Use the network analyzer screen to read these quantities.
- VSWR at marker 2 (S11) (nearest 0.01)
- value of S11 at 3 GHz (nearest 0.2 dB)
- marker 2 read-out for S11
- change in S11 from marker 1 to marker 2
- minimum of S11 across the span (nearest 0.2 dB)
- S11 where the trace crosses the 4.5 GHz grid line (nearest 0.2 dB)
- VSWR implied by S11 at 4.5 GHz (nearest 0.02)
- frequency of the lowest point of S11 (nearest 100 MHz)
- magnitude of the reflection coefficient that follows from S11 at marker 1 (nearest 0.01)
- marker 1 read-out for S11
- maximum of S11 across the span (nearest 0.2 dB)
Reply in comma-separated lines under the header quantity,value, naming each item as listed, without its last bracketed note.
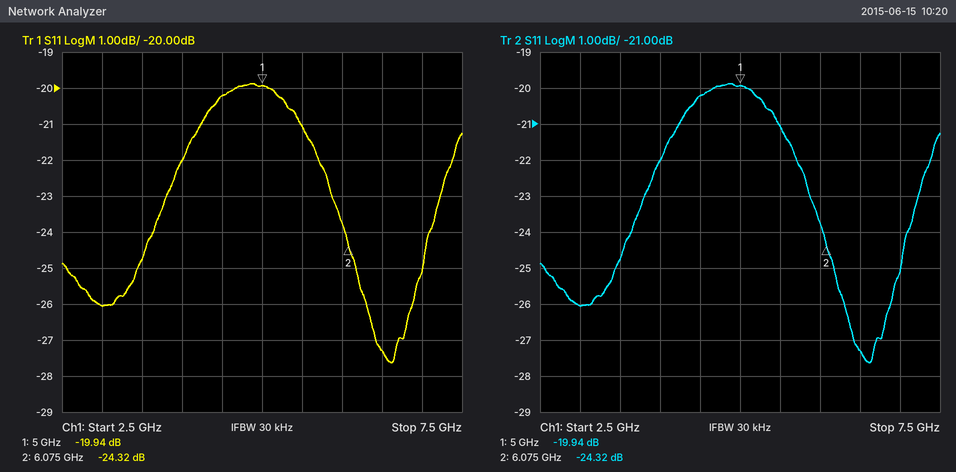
quantity,value
VSWR at marker 2 (S11),1.13
value of S11 at 3 GHz,-26.0 dB
marker 2 read-out for S11,-24.32 dB
change in S11 from marker 1 to marker 2,-4.38 dB
minimum of S11 across the span,-27.6 dB
S11 where the trace crosses the 4.5 GHz grid line,-20.2 dB
VSWR implied by S11 at 4.5 GHz,1.22
frequency of the lowest point of S11,6.6 GHz
magnitude of the reflection coefficient that follows from S11 at marker 1,0.10
marker 1 read-out for S11,-19.94 dB
maximum of S11 across the span,-19.8 dB
